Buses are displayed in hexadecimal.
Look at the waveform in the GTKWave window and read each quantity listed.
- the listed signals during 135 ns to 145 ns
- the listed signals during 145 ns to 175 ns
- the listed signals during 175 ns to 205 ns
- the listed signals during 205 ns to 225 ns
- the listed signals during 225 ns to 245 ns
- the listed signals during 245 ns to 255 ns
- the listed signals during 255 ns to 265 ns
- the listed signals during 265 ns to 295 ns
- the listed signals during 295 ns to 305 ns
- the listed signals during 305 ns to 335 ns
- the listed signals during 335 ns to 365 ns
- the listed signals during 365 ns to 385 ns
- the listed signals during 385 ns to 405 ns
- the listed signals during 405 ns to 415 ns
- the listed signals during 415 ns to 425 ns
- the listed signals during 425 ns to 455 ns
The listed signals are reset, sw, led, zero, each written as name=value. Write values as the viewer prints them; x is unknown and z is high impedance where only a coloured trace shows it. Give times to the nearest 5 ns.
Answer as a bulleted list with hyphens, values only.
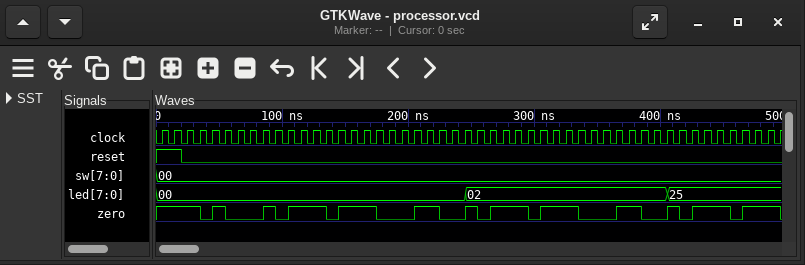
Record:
- reset=0, sw=00, led=00, zero=0
- reset=0, sw=00, led=00, zero=1
- reset=0, sw=00, led=00, zero=0
- reset=0, sw=00, led=00, zero=1
- reset=0, sw=00, led=00, zero=0
- reset=0, sw=00, led=02, zero=1
- reset=0, sw=00, led=02, zero=0
- reset=0, sw=00, led=02, zero=1
- reset=0, sw=00, led=02, zero=0
- reset=0, sw=00, led=02, zero=1
- reset=0, sw=00, led=02, zero=0
- reset=0, sw=00, led=02, zero=1
- reset=0, sw=00, led=02, zero=0
- reset=0, sw=00, led=25, zero=1
- reset=0, sw=00, led=25, zero=0
- reset=0, sw=00, led=25, zero=1
